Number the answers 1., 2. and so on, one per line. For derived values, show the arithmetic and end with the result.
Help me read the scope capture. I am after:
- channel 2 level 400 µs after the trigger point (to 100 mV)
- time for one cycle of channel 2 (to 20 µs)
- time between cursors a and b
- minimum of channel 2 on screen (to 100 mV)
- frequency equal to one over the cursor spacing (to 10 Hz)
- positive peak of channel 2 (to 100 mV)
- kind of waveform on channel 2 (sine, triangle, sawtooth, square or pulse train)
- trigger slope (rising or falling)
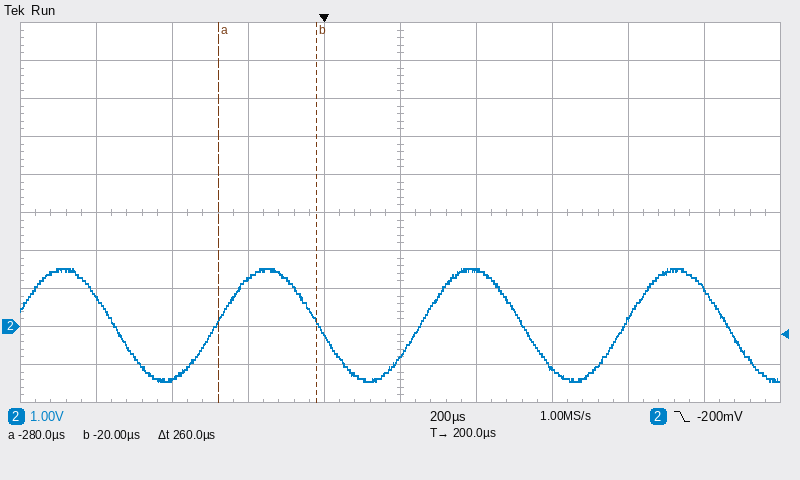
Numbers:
1. 1.5 V
2. 540 µs
3. 260 µs
4. -1.4 V
5. 1 / 260 µs ≈ 3.85 kHz
6. 1.5 V
7. sine
8. falling
